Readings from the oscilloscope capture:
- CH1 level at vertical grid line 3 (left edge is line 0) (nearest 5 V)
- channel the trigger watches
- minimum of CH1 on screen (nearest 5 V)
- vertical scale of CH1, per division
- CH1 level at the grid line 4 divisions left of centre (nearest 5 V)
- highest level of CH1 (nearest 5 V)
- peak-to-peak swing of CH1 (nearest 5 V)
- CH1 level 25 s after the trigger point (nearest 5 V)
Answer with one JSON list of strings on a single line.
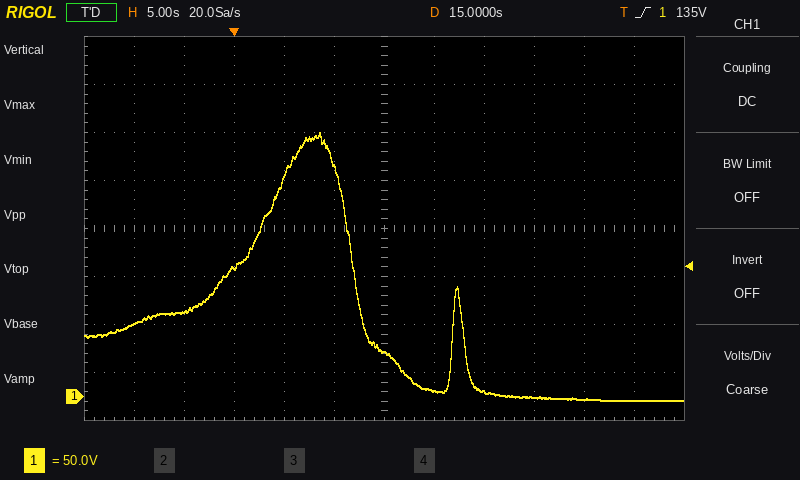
["135 V", "CH1", "-5 V", "50 V", "90 V", "275 V", "280 V", "5 V"]
